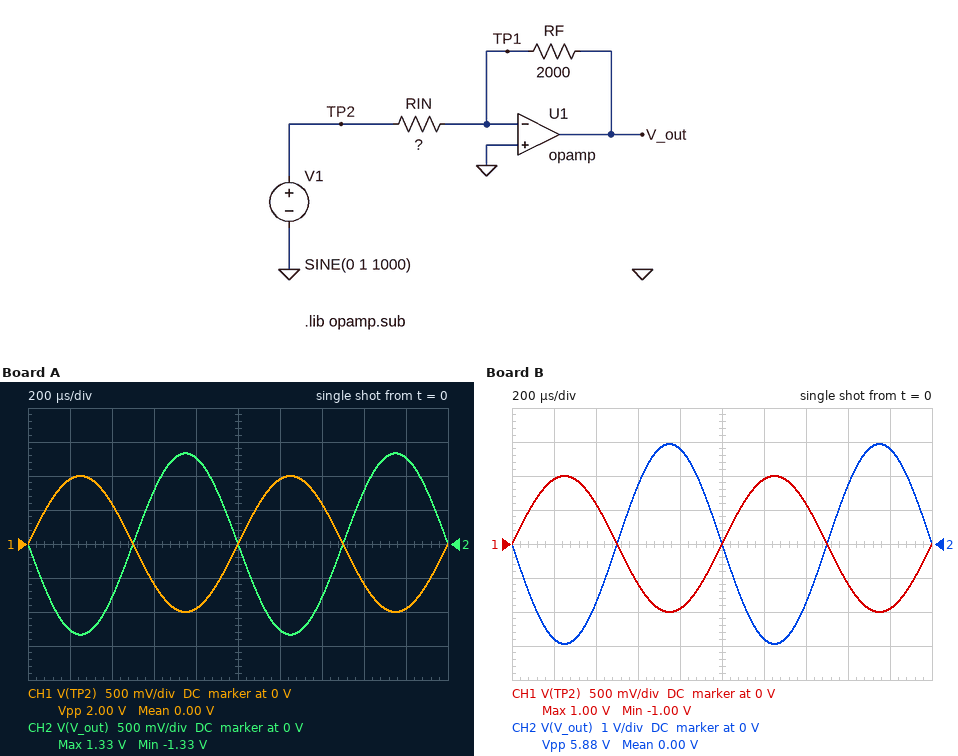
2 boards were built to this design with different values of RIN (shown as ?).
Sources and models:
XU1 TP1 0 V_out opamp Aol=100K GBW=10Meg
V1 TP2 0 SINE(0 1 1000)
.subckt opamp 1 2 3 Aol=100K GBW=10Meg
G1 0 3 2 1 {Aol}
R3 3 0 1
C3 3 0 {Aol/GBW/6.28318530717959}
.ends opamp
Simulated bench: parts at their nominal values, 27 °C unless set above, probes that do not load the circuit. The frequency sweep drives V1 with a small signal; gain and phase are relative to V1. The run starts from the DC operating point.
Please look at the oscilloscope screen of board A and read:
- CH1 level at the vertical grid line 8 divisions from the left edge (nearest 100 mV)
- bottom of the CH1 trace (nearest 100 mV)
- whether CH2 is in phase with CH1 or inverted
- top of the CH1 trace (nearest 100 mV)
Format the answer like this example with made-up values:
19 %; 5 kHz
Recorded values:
-600 mV; -1.0 V; inverted; 1.0 V
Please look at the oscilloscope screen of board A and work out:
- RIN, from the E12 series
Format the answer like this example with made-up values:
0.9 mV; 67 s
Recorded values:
1.5 kΩ
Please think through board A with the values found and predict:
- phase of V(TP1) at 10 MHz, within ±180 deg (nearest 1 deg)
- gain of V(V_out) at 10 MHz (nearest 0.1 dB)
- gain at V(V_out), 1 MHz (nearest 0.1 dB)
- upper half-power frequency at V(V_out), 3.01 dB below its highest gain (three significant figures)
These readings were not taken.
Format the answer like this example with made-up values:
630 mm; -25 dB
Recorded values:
23 deg; -5.6 dB; 2.3 dB; 4.29 MHz
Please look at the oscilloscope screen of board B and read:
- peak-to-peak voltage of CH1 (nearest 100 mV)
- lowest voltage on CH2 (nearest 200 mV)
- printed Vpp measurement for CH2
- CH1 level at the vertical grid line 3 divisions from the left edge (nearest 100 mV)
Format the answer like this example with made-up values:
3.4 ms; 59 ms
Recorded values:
2.0 V; -3.0 V; 5.88 V; -600 mV
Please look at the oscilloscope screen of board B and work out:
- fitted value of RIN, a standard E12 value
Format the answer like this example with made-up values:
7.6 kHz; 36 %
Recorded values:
680 Ω
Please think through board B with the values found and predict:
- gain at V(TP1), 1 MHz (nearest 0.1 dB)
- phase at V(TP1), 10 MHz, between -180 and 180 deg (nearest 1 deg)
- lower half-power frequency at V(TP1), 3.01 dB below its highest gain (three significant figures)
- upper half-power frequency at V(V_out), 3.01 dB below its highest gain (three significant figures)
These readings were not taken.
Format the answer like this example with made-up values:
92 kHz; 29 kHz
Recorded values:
-11.3 dB; 14 deg; 2.54 MHz; 2.54 MHz
